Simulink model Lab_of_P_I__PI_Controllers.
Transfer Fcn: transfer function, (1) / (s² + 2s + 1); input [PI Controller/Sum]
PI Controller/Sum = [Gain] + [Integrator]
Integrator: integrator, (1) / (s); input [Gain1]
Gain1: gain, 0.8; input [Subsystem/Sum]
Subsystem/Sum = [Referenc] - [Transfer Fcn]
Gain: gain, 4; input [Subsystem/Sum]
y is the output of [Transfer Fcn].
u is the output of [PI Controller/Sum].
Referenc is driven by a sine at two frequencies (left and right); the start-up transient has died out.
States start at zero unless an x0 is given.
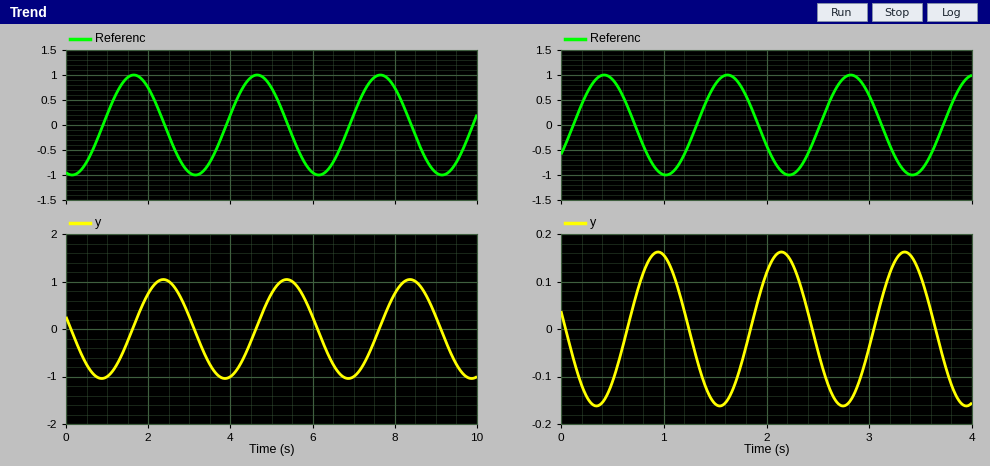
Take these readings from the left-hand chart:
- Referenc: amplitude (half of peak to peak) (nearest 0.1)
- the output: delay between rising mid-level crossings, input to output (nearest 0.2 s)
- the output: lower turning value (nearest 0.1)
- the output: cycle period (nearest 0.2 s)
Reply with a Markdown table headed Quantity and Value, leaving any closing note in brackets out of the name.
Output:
| Quantity | Value |
|---|---|
| Referenc: amplitude (half of peak to peak) | 1.0 |
| the output: delay between rising mid-level crossings, input to output | 0.8 s |
| the output: lower turning value | -1.0 |
| the output: cycle period | 3.0 s |
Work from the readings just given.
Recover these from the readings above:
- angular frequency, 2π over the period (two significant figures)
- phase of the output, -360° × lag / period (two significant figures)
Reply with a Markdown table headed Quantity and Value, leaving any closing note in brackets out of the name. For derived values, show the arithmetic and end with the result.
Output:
| Quantity | Value |
|---|---|
| angular frequency, 2π over the period | 2π / 3 = 2.1 rad/s |
| phase of the output, -360° × lag / period | -360 × 0.8 / 3 = -96° |
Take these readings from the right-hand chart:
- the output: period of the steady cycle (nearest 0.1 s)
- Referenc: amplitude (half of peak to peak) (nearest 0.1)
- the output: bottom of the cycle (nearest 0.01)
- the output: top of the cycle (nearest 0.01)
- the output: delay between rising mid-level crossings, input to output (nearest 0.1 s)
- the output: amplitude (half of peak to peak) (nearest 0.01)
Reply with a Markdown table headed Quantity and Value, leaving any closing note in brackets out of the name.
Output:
| Quantity | Value |
|---|---|
| the output: period of the steady cycle | 1.2 s |
| Referenc: amplitude (half of peak to peak) | 1.0 |
| the output: bottom of the cycle | -0.16 |
| the output: top of the cycle | 0.16 |
| the output: delay between rising mid-level crossings, input to output | 0.5 s |
| the output: amplitude (half of peak to peak) | 0.16 |
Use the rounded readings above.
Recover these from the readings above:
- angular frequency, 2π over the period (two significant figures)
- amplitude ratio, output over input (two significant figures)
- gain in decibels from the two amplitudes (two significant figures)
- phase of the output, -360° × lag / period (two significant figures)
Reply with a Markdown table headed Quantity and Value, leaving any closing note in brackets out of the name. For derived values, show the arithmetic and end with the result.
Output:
| Quantity | Value |
|---|---|
| angular frequency, 2π over the period | 2π / 1.2 = 5.2 rad/s |
| amplitude ratio, output over input | 0.16 / 1 = 0.16 |
| gain in decibels from the two amplitudes | 20 log10(0.16 / 1) = -16 dB |
| phase of the output, -360° × lag / period | -360 × 0.5 / 1.2 = -150° |
